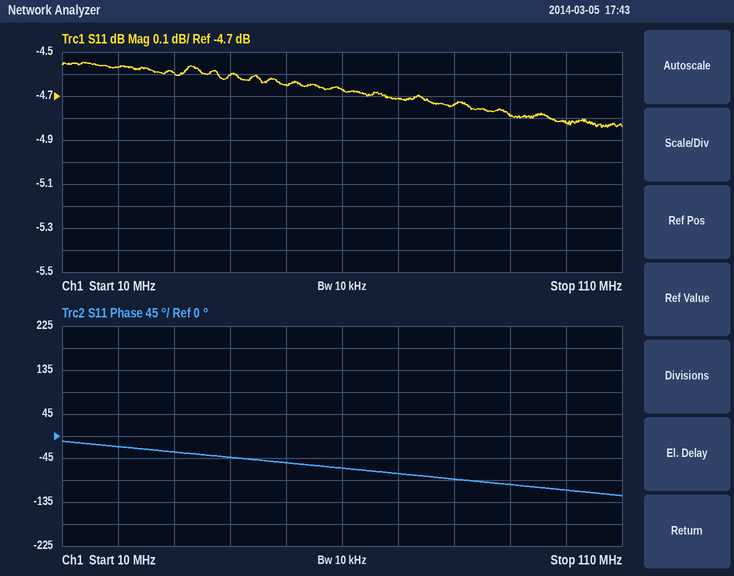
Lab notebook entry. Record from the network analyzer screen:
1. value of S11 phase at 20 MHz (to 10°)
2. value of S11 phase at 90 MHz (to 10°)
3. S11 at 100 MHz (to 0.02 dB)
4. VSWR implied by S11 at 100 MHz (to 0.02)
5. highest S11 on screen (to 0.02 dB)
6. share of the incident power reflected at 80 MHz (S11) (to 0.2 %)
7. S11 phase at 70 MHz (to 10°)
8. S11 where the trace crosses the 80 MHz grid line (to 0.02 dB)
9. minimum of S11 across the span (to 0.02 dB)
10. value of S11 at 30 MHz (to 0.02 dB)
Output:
-20°
-100°
-4.82 dB
3.70
-4.54 dB
33.6 %
-80°
-4.74 dB
-4.84 dB
-4.60 dB
